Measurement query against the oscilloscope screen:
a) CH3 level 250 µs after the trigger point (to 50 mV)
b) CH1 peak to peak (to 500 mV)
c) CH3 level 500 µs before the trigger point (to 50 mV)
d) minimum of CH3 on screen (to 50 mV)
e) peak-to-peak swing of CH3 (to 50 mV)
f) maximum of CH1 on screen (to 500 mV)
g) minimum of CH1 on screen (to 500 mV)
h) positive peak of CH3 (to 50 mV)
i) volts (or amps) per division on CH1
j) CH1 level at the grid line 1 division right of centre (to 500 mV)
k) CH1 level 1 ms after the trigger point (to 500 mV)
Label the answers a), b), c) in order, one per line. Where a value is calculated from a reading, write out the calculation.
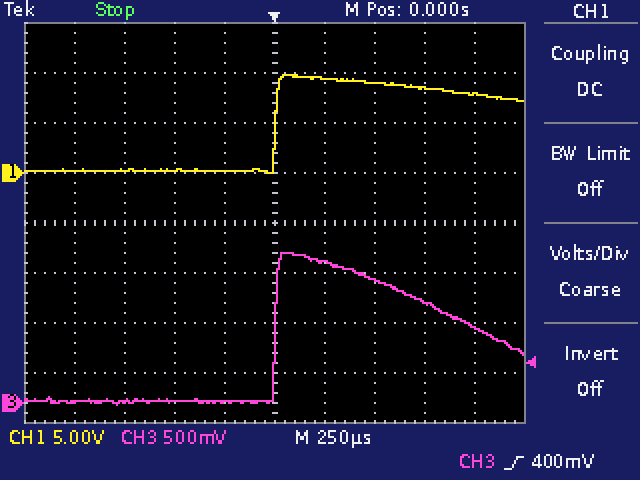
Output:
a) 1.40 V
b) 10.0 V − (0.0 V) = 10.0 V
c) 0 mV
d) 0 mV
e) 1.50 V − (0 mV) = 1.50 V
f) 10.0 V
g) 0.0 V
h) 1.50 V
i) 5 V
j) 9.5 V
k) 8.0 V
